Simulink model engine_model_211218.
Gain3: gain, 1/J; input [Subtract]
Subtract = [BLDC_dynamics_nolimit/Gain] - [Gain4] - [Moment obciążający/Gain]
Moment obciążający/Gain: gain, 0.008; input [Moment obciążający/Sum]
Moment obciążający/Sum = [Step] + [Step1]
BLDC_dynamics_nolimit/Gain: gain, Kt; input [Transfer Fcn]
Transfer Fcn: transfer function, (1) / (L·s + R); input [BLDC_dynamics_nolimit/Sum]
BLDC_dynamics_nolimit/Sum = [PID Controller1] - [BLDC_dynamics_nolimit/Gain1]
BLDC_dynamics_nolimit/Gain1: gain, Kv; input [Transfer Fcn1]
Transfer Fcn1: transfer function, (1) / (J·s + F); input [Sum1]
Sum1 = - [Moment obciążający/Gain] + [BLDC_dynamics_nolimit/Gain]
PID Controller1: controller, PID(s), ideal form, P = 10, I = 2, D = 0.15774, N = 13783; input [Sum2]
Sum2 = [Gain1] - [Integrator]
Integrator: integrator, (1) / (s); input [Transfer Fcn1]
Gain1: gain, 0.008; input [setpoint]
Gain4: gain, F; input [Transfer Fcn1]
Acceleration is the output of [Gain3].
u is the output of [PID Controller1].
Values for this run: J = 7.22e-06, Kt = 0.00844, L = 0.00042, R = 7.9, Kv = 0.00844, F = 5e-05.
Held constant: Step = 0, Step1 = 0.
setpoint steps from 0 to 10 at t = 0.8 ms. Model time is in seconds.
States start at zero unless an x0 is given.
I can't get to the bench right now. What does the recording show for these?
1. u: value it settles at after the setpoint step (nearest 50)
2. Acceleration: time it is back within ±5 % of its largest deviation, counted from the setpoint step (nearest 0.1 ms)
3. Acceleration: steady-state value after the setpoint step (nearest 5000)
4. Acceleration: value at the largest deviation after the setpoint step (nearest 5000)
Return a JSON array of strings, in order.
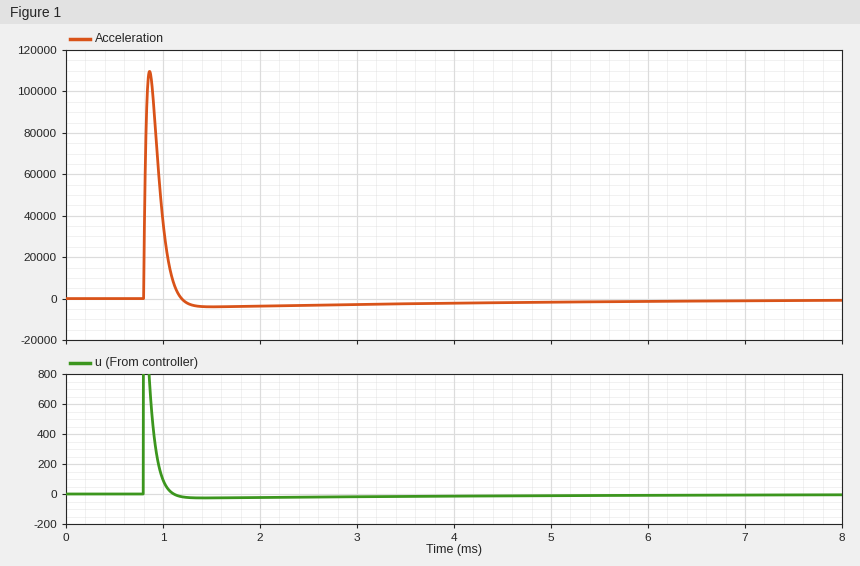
["0", "0.3 ms", "0", "110000"]
